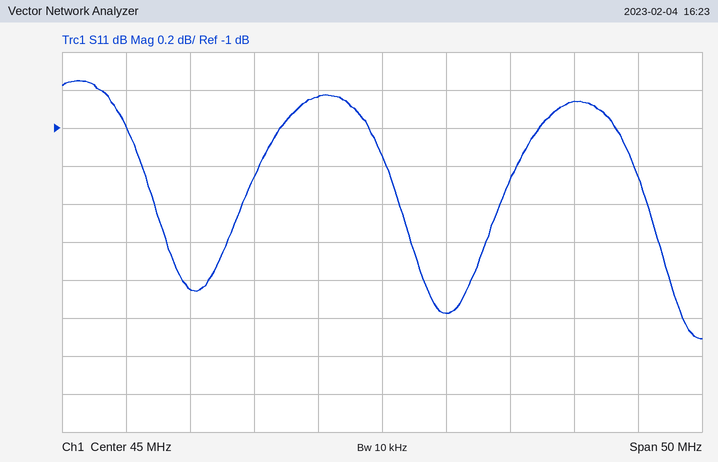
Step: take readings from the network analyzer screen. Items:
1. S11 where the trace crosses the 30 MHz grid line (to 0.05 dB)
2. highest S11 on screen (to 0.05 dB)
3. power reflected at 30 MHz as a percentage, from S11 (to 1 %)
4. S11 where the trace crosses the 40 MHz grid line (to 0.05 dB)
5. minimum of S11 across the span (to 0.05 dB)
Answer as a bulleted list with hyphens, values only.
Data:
- -1.85 dB
- -0.75 dB
- 65 %
- -0.85 dB
- -2.10 dB
